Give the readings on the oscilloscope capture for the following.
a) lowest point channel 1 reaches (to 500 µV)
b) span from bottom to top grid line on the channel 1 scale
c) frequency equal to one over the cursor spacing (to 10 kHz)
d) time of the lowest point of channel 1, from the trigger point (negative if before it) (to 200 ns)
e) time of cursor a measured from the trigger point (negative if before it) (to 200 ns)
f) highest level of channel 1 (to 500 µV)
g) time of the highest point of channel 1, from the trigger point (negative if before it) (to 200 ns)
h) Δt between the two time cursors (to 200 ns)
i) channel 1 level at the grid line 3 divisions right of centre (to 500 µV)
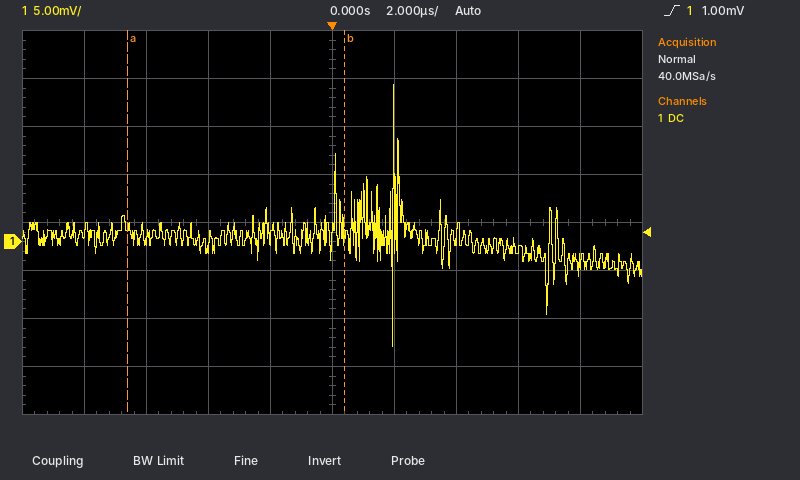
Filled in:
-11.0 mV
40 mV
140 kHz
+2.0 µs
-6.6 µs
16.5 mV
+2.0 µs
7.0 µs
-1.0 mV
